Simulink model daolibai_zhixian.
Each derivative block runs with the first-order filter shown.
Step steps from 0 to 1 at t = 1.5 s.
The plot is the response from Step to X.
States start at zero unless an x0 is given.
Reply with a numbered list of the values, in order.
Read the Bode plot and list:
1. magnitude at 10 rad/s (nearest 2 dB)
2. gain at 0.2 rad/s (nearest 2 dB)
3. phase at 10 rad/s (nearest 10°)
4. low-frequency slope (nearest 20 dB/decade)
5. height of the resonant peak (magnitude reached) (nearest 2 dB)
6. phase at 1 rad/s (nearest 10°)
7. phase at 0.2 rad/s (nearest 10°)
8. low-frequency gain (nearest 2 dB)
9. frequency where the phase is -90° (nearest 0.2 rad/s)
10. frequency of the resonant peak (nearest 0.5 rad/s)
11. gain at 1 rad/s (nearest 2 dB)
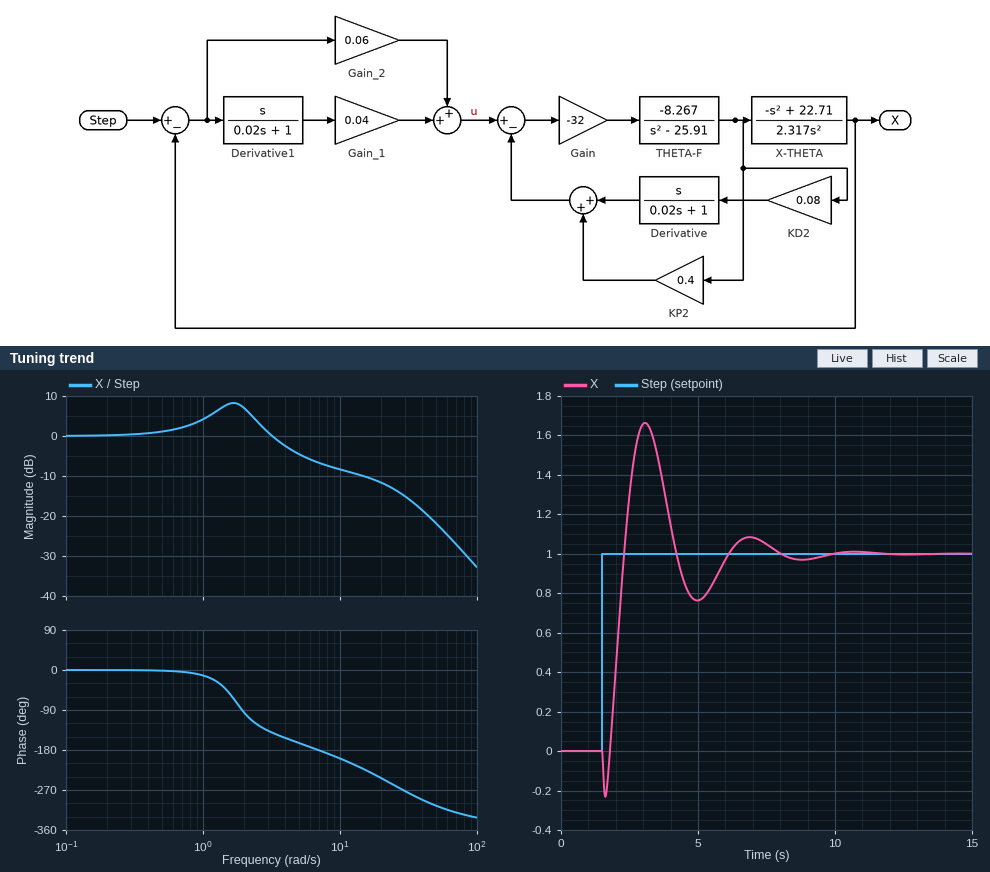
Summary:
1. -8 dB
2. 0 dB
3. -200°
4. 0 dB/decade
5. 8 dB
6. -10°
7. 0°
8. 0 dB
9. 2.0 rad/s
10. 1.5 rad/s
11. 4 dB
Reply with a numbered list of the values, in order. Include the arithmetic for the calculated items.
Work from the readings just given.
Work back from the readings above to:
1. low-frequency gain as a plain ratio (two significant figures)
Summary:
1. 10^(0 / 20) = 1.0
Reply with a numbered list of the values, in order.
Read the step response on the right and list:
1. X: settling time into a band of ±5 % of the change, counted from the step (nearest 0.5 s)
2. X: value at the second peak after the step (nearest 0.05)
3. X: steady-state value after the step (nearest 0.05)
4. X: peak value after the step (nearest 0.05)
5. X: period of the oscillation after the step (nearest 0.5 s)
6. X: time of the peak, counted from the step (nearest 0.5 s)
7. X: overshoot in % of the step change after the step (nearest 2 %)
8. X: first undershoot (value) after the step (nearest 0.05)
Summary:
1. 6.0 s
2. 1.10
3. 1.00
4. 1.65
5. 4.0 s
6. 1.5 s
7. 66 %
8. 0.75
